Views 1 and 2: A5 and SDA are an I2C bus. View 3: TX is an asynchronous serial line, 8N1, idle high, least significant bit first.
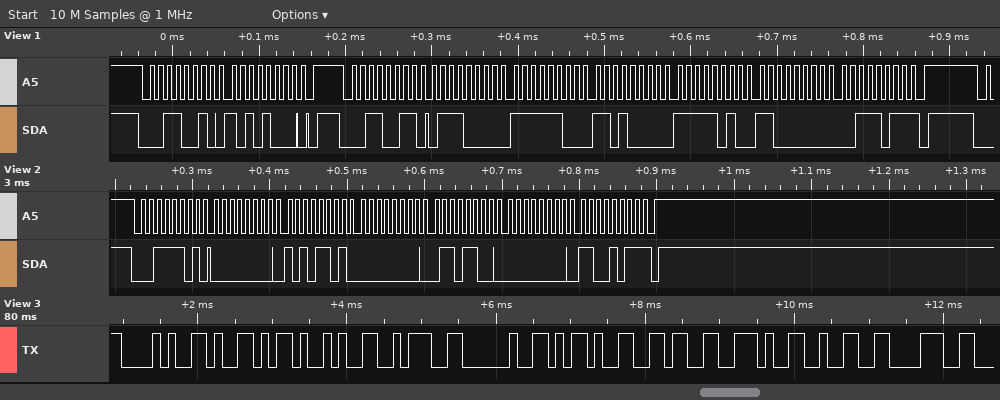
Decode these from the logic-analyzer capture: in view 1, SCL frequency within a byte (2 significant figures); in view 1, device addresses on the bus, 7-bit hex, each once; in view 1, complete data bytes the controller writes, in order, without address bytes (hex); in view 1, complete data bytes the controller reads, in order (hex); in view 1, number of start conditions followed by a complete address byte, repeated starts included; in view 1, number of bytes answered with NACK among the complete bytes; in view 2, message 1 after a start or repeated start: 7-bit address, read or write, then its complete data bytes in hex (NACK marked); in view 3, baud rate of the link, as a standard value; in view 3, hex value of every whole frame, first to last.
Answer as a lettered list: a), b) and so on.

a) 100 kHz
b) 0x19
c) A8
d) 70 FC D0 FA C0 3B
e) 2
f) 1
g) 0x1E read: 00 AD 00 6C 00 CB NACK
h) 9600 baud
i) 28 59 29 3A 20 2D 36 2E 32 38
